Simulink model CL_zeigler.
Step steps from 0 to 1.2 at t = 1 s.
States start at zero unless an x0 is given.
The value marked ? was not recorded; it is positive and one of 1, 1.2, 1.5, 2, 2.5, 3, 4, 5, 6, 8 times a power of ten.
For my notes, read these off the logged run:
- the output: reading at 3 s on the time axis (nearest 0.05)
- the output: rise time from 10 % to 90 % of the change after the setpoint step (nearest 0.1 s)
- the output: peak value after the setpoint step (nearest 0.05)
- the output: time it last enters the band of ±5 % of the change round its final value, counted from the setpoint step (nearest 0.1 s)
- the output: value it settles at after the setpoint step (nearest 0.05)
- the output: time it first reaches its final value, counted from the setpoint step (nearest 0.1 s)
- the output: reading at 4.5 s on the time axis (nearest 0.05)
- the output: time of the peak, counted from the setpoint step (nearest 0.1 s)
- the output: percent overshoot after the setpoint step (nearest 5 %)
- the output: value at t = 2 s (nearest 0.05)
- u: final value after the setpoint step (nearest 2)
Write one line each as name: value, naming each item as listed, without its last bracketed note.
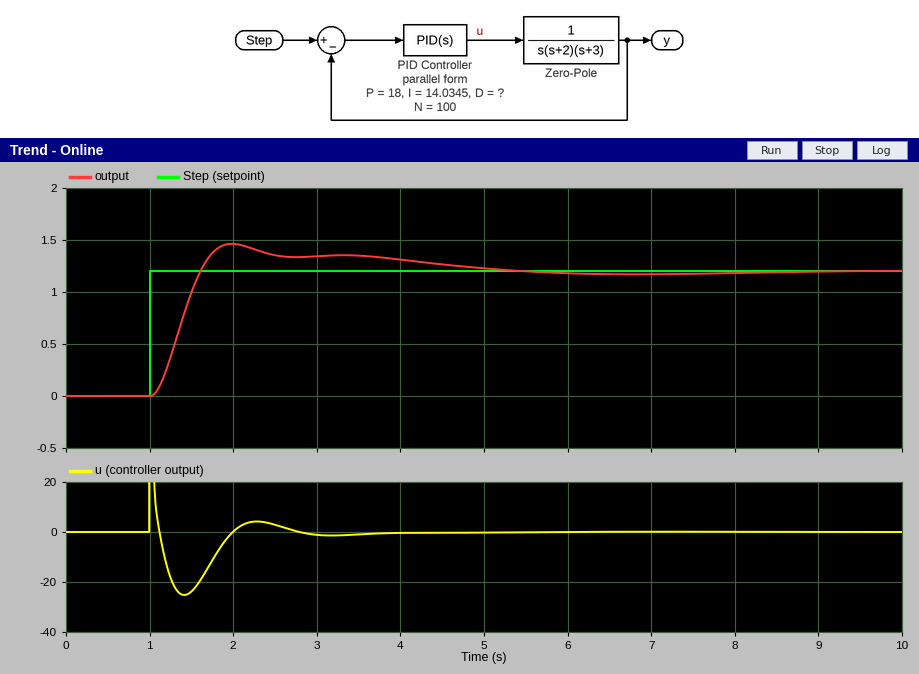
the output: reading at 3 s on the time axis: 1.35
the output: rise time from 10 % to 90 % of the change after the setpoint step: 0.4 s
the output: peak value after the setpoint step: 1.45
the output: time it last enters the band of ±5 % of the change round its final value, counted from the setpoint step: 3.6 s
the output: value it settles at after the setpoint step: 1.20
the output: time it first reaches its final value, counted from the setpoint step: 0.6 s
the output: reading at 4.5 s on the time axis: 1.25
the output: time of the peak, counted from the setpoint step: 1.0 s
the output: percent overshoot after the setpoint step: 20 %
the output: value at t = 2 s: 1.45
u: final value after the setpoint step: 0
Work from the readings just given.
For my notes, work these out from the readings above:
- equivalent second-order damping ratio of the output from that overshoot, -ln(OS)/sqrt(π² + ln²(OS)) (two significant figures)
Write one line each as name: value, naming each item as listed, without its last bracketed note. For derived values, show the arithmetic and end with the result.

equivalent second-order damping ratio of the output from that overshoot, -ln(OS)/sqrt(π² + ln²(OS)): ln(0.2) = -1.609; 1.609 / sqrt(9.870 + 2.590) = 0.46
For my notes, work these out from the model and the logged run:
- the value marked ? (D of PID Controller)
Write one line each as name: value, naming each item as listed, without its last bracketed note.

the value marked ?: 15
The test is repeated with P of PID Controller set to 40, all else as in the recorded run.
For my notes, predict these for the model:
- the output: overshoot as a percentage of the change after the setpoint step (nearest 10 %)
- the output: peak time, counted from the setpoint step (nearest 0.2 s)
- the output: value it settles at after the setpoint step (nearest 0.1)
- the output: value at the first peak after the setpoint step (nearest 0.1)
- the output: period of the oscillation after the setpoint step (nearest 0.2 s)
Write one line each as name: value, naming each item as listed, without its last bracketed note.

the output: overshoot as a percentage of the change after the setpoint step: 50 %
the output: peak time, counted from the setpoint step: 0.8 s
the output: value it settles at after the setpoint step: 1.2
the output: value at the first peak after the setpoint step: 1.8
the output: period of the oscillation after the setpoint step: 1.8 s
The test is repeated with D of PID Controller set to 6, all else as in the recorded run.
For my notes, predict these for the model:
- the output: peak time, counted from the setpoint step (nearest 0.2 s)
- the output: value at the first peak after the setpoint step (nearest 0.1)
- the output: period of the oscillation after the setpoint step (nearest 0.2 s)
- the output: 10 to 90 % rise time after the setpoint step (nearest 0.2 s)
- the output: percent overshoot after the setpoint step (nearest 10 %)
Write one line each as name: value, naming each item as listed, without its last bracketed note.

the output: peak time, counted from the setpoint step: 1.6 s
the output: value at the first peak after the setpoint step: 1.9
the output: period of the oscillation after the setpoint step: 3.6 s
the output: 10 to 90 % rise time after the setpoint step: 0.6 s
the output: percent overshoot after the setpoint step: 60 %
